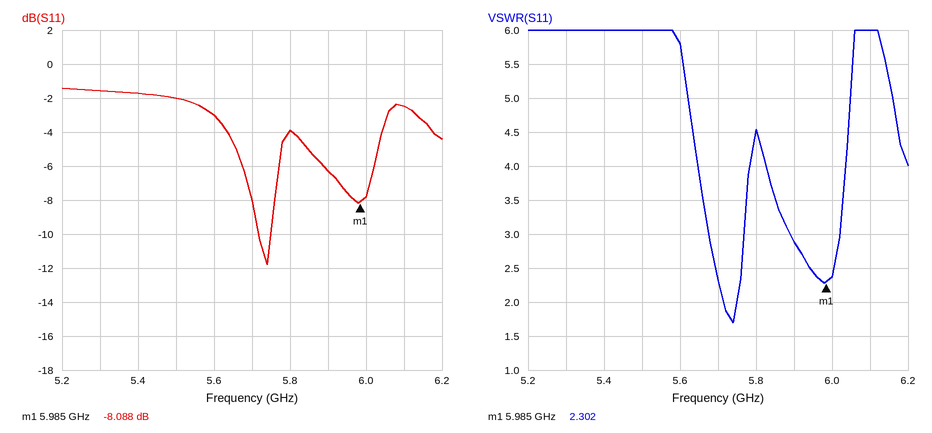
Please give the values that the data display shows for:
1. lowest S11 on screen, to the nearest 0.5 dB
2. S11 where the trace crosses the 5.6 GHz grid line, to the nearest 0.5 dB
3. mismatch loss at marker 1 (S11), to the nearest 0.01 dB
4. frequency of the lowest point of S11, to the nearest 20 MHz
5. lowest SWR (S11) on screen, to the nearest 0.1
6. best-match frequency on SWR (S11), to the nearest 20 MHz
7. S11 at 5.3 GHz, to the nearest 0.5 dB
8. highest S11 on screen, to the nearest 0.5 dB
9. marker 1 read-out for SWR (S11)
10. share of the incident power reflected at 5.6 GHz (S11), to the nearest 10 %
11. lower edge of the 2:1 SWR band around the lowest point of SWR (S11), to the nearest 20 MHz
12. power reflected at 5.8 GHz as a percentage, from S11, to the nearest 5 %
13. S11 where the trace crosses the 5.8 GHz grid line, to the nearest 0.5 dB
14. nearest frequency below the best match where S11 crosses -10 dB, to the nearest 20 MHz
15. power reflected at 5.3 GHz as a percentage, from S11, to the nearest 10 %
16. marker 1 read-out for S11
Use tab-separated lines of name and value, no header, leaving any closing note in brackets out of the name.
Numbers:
lowest S11 on screen, to the nearest 0.5 dB	-12.0 dB
S11 where the trace crosses the 5.6 GHz grid line, to the nearest 0.5 dB	-3.0 dB
mismatch loss at marker 1 (S11), to the nearest 0.01 dB	0.73 dB
frequency of the lowest point of S11, to the nearest 20 MHz	5.74 GHz
lowest SWR (S11) on screen, to the nearest 0.1	1.7
best-match frequency on SWR (S11), to the nearest 20 MHz	5.74 GHz
S11 at 5.3 GHz, to the nearest 0.5 dB	-1.5 dB
highest S11 on screen, to the nearest 0.5 dB	-1.5 dB
marker 1 read-out for SWR	2.302
share of the incident power reflected at 5.6 GHz (S11), to the nearest 10 %	50 %
lower edge of the 2:1 SWR band around the lowest point of SWR (S11), to the nearest 20 MHz	5.72 GHz
power reflected at 5.8 GHz as a percentage, from S11, to the nearest 5 %	40 %
S11 where the trace crosses the 5.8 GHz grid line, to the nearest 0.5 dB	-4.0 dB
nearest frequency below the best match where S11 crosses -10 dB, to the nearest 20 MHz	5.72 GHz
power reflected at 5.3 GHz as a percentage, from S11, to the nearest 10 %	70 %
marker 1 read-out for S11	-8.088 dB
